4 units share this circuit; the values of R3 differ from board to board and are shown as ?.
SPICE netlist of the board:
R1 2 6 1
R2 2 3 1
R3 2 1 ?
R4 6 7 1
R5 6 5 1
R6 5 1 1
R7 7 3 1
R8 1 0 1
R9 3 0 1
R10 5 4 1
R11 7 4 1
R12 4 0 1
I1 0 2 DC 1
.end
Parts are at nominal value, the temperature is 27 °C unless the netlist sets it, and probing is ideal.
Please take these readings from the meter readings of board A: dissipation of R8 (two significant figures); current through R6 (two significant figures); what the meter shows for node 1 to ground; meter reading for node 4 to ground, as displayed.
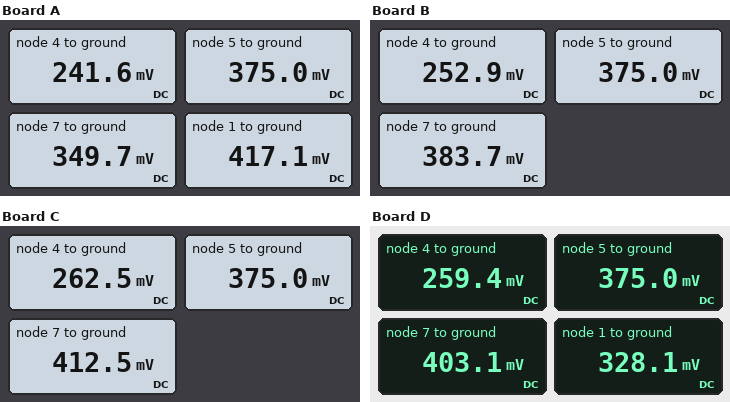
170 mW
42 mA
417.1 mV
241.6 mV
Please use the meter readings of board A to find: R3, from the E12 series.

0.56 Ω
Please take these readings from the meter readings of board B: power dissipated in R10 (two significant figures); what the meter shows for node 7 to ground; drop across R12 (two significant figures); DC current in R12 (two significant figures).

15 mW
383.7 mV
250 mV
250 mA
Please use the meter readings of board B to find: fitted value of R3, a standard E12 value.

1.2 Ω
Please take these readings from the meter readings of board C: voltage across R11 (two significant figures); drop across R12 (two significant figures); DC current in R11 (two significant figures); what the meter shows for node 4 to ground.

150 mV
260 mV
150 mA
262.5 mV
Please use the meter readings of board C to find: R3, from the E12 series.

2.2 Ω
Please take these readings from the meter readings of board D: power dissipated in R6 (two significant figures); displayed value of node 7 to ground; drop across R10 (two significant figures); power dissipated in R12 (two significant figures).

2.2 mW
403.1 mV
120 mV
67 mW
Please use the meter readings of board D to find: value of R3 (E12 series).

1.8 Ω
